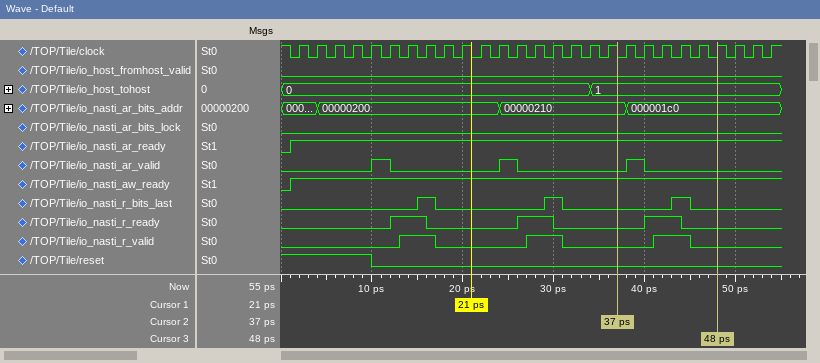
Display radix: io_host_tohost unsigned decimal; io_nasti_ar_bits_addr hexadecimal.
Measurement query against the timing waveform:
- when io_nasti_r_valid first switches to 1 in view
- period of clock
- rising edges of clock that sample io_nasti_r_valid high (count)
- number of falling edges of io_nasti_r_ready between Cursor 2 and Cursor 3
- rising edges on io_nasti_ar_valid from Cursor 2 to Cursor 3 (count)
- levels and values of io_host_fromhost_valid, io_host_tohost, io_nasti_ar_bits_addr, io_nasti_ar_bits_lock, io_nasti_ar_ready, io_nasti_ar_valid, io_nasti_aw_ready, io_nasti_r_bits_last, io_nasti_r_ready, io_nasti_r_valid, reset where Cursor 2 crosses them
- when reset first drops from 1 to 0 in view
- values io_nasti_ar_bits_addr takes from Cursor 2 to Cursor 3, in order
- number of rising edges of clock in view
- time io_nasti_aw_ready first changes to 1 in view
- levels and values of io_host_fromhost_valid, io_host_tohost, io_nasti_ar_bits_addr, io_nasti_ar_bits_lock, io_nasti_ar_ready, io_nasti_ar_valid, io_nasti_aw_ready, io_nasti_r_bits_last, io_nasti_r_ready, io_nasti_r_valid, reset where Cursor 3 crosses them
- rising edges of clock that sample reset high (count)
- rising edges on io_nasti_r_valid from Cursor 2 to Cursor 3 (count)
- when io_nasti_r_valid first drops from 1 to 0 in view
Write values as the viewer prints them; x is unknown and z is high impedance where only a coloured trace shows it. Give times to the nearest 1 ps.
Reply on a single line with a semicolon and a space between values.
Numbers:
13 ps; 2 ps; 6; 1; 1; io_host_fromhost_valid=0, io_host_tohost=1, io_nasti_ar_bits_addr=00000210, io_nasti_ar_bits_lock=0, io_nasti_ar_ready=1, io_nasti_ar_valid=0, io_nasti_aw_ready=1, io_nasti_r_bits_last=0, io_nasti_r_ready=0, io_nasti_r_valid=0, reset=0; 10 ps; 00000210, 000001c0; 27; 1 ps; io_host_fromhost_valid=0, io_host_tohost=1, io_nasti_ar_bits_addr=000001c0, io_nasti_ar_bits_lock=0, io_nasti_ar_ready=1, io_nasti_ar_valid=0, io_nasti_aw_ready=1, io_nasti_r_bits_last=0, io_nasti_r_ready=0, io_nasti_r_valid=0, reset=0; 5; 1; 17 ps
